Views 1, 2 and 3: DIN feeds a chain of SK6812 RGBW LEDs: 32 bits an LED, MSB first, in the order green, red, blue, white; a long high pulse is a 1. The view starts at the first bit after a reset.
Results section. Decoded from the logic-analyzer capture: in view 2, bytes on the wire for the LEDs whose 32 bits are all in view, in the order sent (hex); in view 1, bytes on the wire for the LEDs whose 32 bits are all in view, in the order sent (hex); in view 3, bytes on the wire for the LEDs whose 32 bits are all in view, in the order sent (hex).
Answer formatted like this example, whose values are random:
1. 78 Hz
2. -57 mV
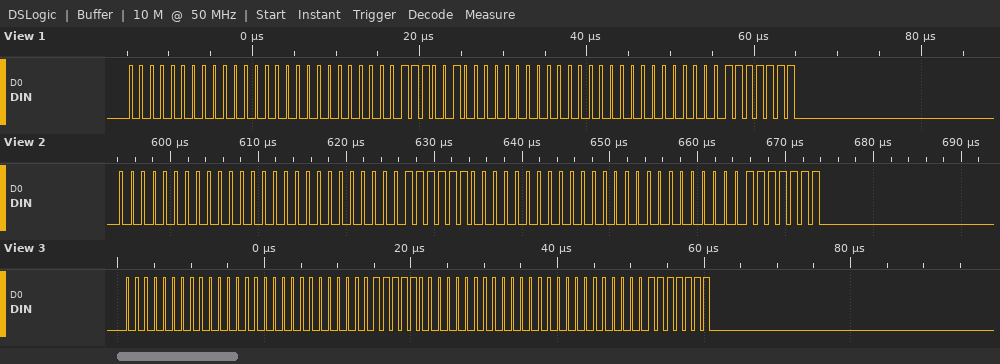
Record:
1. 00 00 00 3F 00 00 00 7F
2. 00 00 00 39 00 00 00 7F
3. 00 00 00 1F 00 00 00 7F
